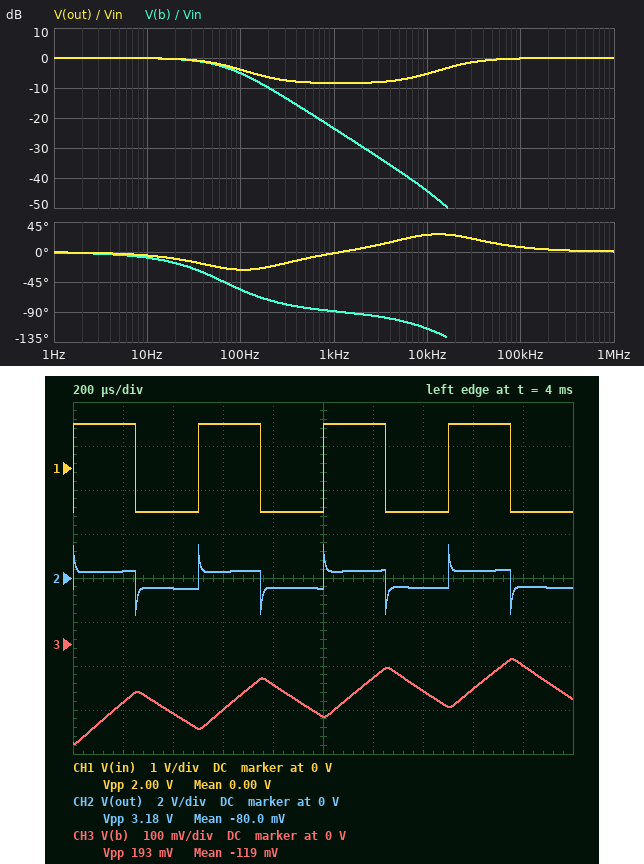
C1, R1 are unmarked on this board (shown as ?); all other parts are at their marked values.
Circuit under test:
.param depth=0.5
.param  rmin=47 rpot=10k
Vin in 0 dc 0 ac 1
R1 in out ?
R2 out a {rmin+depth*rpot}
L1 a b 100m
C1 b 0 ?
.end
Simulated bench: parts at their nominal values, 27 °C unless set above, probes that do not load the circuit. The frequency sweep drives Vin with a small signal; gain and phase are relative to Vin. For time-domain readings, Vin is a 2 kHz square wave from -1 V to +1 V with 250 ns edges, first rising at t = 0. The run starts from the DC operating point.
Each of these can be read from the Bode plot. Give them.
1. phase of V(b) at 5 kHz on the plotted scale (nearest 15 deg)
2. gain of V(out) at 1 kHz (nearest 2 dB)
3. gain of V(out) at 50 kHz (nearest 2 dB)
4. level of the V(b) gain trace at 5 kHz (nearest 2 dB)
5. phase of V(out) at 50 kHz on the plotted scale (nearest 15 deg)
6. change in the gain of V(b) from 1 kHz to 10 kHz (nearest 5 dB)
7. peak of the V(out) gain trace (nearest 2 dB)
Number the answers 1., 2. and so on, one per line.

1. -105 deg
2. -8 dB
3. 0 dB
4. -38 dB
5. 15 deg
6. -20 dB
7. 0 dB
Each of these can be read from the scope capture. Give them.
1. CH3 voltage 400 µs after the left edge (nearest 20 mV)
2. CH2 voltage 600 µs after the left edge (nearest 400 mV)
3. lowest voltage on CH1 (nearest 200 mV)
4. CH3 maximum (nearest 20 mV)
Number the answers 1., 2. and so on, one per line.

1. -160 mV
2. 400 mV
3. -1.0 V
4. -40 mV
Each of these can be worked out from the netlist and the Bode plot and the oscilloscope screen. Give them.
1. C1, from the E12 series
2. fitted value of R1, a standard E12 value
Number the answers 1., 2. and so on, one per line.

1. 180 nF
2. 8.2 kΩ
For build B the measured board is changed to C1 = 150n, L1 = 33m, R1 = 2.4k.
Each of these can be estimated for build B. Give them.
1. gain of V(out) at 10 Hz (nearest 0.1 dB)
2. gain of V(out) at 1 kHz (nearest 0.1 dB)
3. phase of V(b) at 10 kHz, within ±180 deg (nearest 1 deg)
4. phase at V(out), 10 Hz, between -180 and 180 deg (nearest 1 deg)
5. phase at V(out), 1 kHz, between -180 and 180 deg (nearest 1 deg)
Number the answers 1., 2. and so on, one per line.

1. 0 dB
2. -3.3 dB
3. -105 deg
4. -1 deg
5. -3 deg
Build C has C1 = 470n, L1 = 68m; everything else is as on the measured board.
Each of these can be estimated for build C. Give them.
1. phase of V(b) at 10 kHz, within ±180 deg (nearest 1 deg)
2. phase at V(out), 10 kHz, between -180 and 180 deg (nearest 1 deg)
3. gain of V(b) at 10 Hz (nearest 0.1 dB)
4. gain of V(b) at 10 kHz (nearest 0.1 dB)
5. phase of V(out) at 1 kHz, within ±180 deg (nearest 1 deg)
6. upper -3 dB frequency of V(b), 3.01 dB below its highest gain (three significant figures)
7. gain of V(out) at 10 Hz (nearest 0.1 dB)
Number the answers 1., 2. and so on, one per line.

1. -108 deg
2. 22 deg
3. -0.6 dB
4. -52.3 dB
5. 1 deg
6. 25.6 Hz
7. -0.5 dB
